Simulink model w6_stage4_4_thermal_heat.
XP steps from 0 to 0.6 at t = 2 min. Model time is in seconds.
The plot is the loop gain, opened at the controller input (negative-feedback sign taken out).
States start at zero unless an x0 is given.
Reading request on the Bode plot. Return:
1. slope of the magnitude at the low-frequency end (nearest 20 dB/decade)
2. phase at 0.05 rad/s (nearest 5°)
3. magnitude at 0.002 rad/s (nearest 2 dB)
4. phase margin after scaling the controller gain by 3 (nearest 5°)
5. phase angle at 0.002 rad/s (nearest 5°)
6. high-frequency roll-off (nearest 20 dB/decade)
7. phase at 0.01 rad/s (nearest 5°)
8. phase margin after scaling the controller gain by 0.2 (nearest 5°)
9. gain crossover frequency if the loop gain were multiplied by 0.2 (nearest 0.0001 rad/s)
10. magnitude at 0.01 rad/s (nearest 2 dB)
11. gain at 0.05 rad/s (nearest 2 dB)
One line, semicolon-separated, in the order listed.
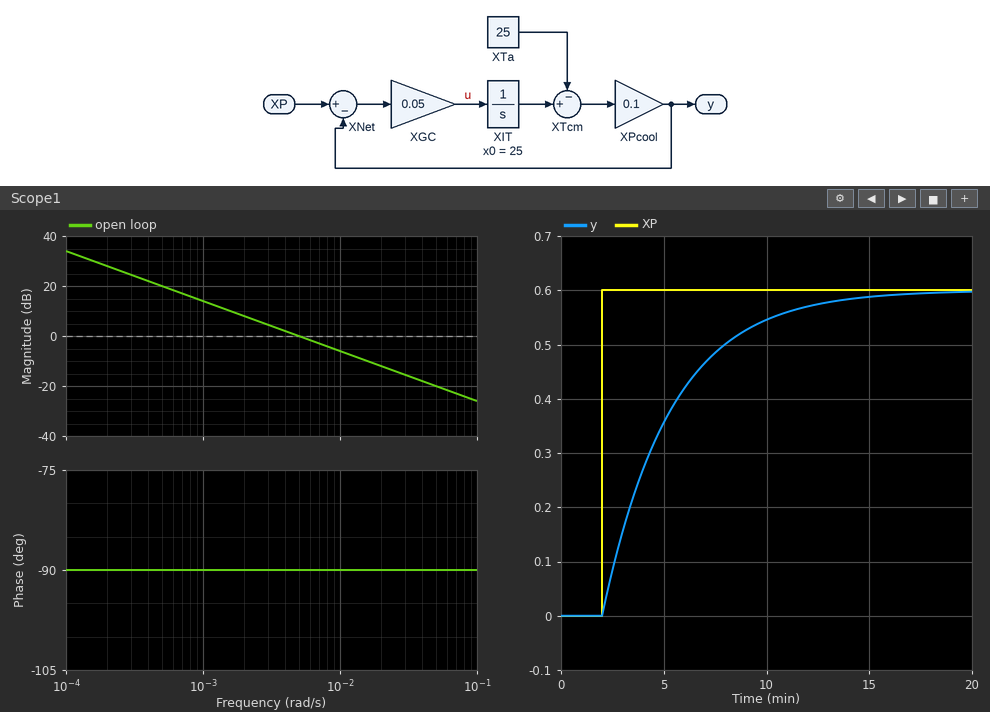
-20 dB/decade; -90°; 8 dB; 90°; -90°; -20 dB/decade; -90°; 90°; 0.0010 rad/s; -6 dB; -20 dB
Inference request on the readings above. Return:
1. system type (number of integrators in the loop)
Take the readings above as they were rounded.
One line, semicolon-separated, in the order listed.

1
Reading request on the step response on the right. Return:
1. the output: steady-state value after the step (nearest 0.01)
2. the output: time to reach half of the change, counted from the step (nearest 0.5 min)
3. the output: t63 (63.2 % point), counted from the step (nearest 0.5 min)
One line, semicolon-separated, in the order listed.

0.60; 2.5 min; 3.5 min
